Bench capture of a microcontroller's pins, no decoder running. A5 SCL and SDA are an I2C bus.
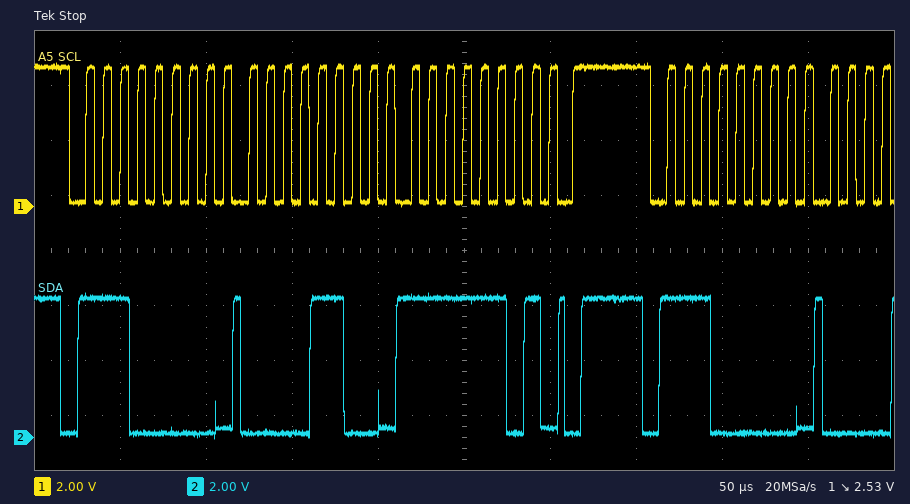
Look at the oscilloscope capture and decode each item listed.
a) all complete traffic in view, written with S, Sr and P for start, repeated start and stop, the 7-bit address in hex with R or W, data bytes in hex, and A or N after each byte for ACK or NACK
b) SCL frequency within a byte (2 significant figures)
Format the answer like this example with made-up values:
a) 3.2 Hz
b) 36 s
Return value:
a) S 70W A 0C A FD A P S 70W A
b) 100 kHz
